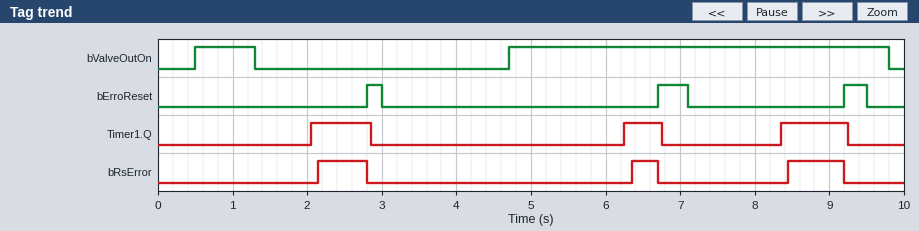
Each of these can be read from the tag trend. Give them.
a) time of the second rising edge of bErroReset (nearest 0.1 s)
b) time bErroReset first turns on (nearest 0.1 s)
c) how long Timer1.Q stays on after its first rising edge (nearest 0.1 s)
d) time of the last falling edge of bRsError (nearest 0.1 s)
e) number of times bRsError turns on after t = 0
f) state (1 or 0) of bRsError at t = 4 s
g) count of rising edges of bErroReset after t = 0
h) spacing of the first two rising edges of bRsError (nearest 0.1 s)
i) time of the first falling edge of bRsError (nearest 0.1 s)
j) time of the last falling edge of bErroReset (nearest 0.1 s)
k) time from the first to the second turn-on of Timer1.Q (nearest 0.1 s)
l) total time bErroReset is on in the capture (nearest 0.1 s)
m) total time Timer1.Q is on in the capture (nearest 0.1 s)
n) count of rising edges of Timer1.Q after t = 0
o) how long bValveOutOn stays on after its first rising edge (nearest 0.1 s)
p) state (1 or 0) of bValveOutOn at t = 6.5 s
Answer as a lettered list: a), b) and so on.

a) 6.7 s
b) 2.8 s
c) 0.8 s
d) 9.2 s
e) 3
f) 0
g) 3
h) 4.2 s
i) 2.8 s
j) 9.5 s
k) 4.2 s
l) 0.9 s
m) 2.2 s
n) 3
o) 0.8 s
p) 1
